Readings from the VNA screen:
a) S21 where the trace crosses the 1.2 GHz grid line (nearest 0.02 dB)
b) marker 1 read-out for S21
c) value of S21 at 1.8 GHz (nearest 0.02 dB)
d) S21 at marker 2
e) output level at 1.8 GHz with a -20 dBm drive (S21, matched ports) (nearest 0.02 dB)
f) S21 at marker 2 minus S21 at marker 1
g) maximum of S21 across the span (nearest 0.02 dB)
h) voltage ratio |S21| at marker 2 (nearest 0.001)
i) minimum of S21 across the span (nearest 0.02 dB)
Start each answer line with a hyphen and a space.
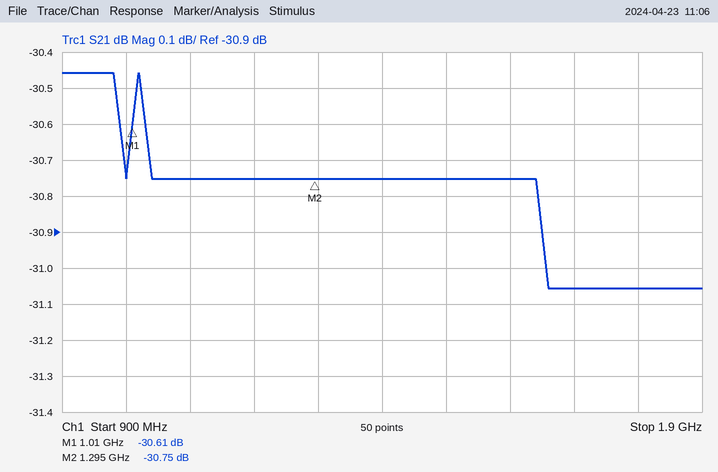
- -30.76 dB
- -30.61 dB
- -31.06 dB
- -30.75 dB
- -51.06 dBm
- -0.14 dB
- -30.46 dB
- 0.029
- -31.06 dB
